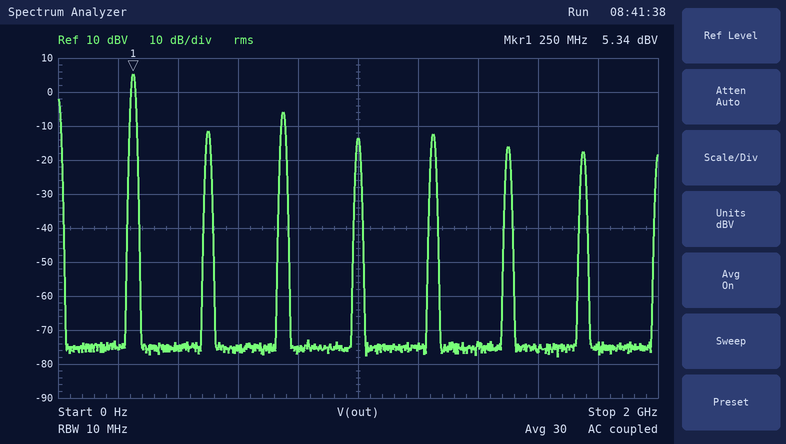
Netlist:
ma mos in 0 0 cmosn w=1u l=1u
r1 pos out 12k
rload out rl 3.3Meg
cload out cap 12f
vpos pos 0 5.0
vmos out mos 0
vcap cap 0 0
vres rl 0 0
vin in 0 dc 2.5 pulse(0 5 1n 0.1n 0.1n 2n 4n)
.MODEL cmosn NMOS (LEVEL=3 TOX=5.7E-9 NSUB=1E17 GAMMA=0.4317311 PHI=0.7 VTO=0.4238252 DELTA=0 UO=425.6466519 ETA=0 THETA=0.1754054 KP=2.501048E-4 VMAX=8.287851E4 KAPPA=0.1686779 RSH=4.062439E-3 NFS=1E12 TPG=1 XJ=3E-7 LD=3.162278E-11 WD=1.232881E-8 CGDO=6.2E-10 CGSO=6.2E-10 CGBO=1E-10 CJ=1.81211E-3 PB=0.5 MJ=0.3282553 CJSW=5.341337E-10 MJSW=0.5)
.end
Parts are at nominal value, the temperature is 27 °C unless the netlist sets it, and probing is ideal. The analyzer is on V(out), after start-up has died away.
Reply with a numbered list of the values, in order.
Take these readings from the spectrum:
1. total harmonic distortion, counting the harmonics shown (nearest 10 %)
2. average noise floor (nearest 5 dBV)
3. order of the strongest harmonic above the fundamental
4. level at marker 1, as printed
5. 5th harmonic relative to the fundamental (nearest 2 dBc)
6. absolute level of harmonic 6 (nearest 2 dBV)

1. 40 %
2. -75 dBV
3. 3
4. 5.34 dBV
5. -18 dBc
6. -16 dBV
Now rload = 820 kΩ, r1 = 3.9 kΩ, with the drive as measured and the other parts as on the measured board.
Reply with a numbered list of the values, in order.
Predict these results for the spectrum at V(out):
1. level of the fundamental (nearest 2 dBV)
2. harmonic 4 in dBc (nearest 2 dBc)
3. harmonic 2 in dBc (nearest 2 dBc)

1. 0 dBV
2. -24 dBc
3. -24 dBc
